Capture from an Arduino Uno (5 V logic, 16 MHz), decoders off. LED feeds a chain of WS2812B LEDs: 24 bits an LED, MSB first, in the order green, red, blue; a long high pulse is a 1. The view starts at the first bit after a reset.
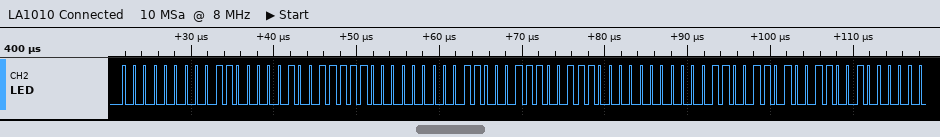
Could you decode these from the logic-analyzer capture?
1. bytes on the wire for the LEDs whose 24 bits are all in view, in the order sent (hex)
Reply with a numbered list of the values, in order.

1. 00 60 9F 00 63 9C 00 66 99
